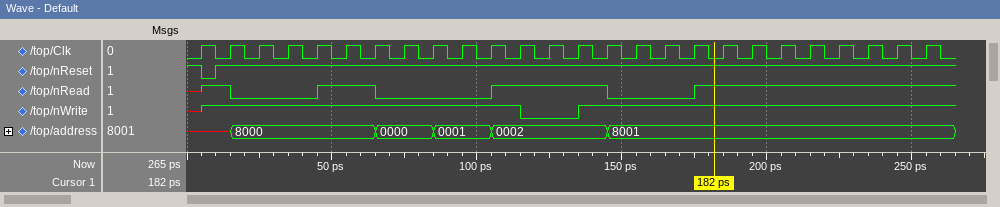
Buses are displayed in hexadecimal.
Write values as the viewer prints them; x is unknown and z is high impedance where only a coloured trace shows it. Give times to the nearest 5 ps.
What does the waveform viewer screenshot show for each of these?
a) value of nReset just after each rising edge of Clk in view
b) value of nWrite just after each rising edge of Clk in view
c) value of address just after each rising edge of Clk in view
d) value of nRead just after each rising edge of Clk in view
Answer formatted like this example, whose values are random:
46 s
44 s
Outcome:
0 1 1 1 1 1 1 1 1 1 1 1 1 1 1 1 1 1 1 1 1 1 1 1 1 1
1 1 1 1 1 1 1 1 1 1 1 0 0 1 1 1 1 1 1 1 1 1 1 1 1 1
x, 8000, 8000, 8000, 8000, 8000, 0000, 0000, 0001, 0001, 0002, 0002, 0002, 0002, 8001, 8001, 8001, 8001, 8001, 8001, 8001, 8001, 8001, 8001, 8001, 8001
1 0 0 0 1 1 0 0 0 0 1 1 1 1 0 0 0 1 1 1 1 1 1 1 1 1
